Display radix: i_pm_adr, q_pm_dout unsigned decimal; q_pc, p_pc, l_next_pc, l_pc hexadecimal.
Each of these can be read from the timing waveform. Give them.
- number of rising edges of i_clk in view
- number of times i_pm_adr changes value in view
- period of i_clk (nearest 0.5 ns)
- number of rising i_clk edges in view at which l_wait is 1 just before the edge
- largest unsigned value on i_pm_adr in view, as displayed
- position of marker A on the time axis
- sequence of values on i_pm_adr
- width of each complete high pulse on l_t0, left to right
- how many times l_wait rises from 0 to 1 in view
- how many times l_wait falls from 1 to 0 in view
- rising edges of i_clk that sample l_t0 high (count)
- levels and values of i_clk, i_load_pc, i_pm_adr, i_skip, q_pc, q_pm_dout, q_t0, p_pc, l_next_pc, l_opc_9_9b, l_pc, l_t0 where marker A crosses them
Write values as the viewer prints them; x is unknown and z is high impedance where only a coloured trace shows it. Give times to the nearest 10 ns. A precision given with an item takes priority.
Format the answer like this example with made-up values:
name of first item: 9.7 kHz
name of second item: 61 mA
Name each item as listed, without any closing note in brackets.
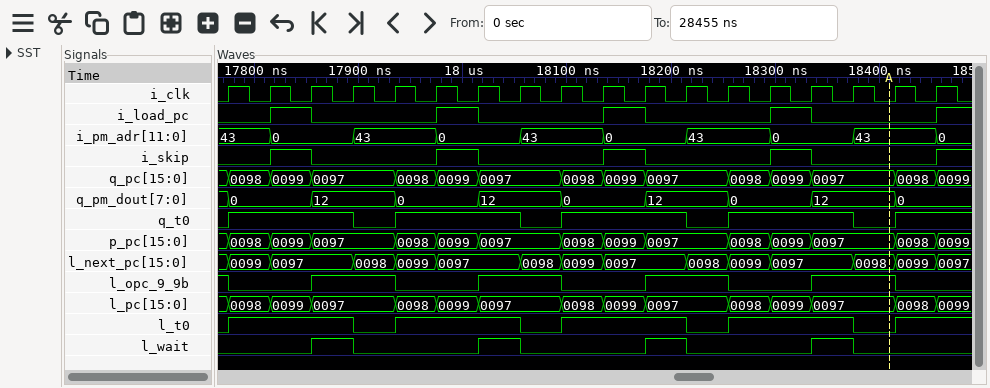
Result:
number of rising edges of i_clk in view: 18
number of times i_pm_adr changes value in view: 9
period of i_clk: 40 ns
number of rising i_clk edges in view at which l_wait is 1 just before the edge: 4
largest unsigned value on i_pm_adr in view, as displayed: 43
position of marker A on the time axis: 18410 ns
sequence of values on i_pm_adr: 43, 0, 43, 0, 43, 0, 43, 0, 43, 0
width of each complete high pulse on l_t0, left to right: 120 ns, 120 ns, 120 ns, 120 ns
how many times l_wait rises from 0 to 1 in view: 4
how many times l_wait falls from 1 to 0 in view: 4
rising edges of i_clk that sample l_t0 high: 13
levels and values of i_clk, i_load_pc, i_pm_adr, i_skip, q_pc, q_pm_dout, q_t0, p_pc, l_next_pc, l_opc_9_9b, l_pc, l_t0 where marker A crosses them: i_clk=0, i_load_pc=0, i_pm_adr=43, i_skip=0, q_pc=0097, q_pm_dout=12, q_t0=0, p_pc=0097, l_next_pc=0098, l_opc_9_9b=1, l_pc=0097, l_t0=0
